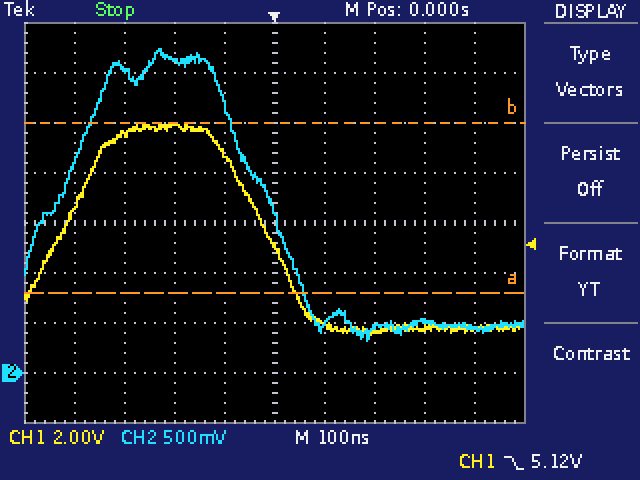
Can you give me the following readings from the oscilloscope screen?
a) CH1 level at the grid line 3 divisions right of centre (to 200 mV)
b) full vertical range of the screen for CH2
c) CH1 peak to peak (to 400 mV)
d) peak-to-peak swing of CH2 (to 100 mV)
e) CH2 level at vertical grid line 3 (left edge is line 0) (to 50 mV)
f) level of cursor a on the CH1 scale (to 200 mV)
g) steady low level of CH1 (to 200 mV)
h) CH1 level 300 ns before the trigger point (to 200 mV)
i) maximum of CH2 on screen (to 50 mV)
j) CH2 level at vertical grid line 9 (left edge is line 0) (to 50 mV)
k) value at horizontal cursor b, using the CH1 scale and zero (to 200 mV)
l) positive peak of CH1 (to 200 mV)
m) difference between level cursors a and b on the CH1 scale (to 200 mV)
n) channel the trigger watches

1.8 V
4 V
8.4 V
2.90 V
3.15 V
3.2 V
1.8 V
9.6 V
3.25 V
450 mV
10.0 V
10.0 V
6.8 V
CH1
